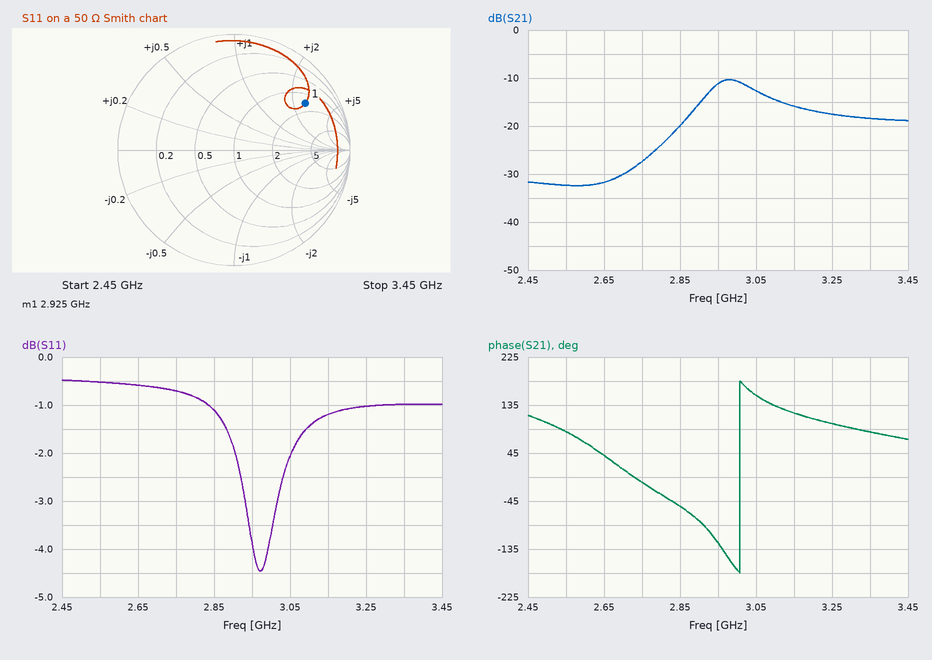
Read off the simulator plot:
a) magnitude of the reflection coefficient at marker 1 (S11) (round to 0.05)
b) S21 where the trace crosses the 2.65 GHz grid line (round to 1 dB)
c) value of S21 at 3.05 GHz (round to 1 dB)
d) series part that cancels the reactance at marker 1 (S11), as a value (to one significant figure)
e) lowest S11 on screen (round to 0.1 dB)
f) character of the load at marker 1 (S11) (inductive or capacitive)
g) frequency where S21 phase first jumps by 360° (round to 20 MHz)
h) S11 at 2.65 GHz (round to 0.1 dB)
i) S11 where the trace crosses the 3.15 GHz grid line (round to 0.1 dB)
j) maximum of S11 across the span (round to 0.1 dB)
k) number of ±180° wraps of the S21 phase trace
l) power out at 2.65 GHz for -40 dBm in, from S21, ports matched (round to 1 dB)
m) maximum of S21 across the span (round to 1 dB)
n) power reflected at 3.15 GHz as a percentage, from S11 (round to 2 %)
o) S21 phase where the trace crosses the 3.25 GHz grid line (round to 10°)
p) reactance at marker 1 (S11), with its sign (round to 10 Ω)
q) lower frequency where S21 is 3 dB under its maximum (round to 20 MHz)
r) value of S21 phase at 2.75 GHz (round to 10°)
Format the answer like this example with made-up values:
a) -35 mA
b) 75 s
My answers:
a) 0.75
b) -32 dB
c) -13 dB
d) 400 fF
e) -4.5 dB
f) inductive
g) 3.00 GHz
h) -0.6 dB
i) -1.2 dB
j) -0.5 dB
k) 1
l) -72 dBm
m) -10 dB
n) 76 %
o) 100°
p) +130 Ω
q) 2.92 GHz
r) -10°
